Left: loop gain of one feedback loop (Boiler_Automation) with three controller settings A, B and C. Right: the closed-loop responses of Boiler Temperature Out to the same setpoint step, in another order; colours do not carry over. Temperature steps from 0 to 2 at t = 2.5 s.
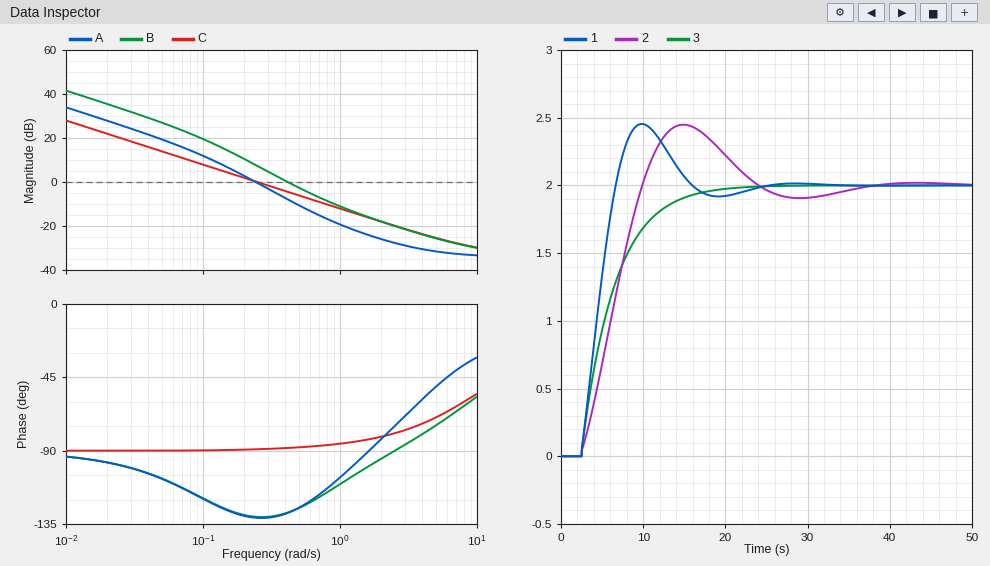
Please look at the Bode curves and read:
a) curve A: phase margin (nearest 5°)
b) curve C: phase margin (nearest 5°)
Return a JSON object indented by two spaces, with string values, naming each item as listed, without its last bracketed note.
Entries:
{
  "curve A: phase margin": "50°",
  "curve C: phase margin": "90°"
}
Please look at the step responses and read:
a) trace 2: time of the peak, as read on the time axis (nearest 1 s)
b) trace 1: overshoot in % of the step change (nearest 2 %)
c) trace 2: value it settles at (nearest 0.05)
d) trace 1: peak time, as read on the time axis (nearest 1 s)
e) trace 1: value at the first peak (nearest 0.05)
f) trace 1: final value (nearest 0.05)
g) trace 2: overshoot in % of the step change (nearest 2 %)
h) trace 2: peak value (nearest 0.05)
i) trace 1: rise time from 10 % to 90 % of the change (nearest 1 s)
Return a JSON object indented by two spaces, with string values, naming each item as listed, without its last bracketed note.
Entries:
{
  "trace 2: time of the peak, as read on the time axis": "15 s",
  "trace 1: overshoot in % of the step change": "22 %",
  "trace 2: value it settles at": "2.00",
  "trace 1: peak time, as read on the time axis": "10 s",
  "trace 1: value at the first peak": "2.45",
  "trace 1: final value": "2.00",
  "trace 2: overshoot in % of the step change": "22 %",
  "trace 2: peak value": "2.45",
  "trace 1: rise time from 10 % to 90 % of the change": "3 s"
}
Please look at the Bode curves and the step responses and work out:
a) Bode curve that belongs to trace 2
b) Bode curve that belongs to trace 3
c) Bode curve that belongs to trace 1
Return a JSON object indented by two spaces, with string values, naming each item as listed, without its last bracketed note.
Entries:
{
  "Bode curve that belongs to trace 2": "A",
  "Bode curve that belongs to trace 3": "C",
  "Bode curve that belongs to trace 1": "B"
}
